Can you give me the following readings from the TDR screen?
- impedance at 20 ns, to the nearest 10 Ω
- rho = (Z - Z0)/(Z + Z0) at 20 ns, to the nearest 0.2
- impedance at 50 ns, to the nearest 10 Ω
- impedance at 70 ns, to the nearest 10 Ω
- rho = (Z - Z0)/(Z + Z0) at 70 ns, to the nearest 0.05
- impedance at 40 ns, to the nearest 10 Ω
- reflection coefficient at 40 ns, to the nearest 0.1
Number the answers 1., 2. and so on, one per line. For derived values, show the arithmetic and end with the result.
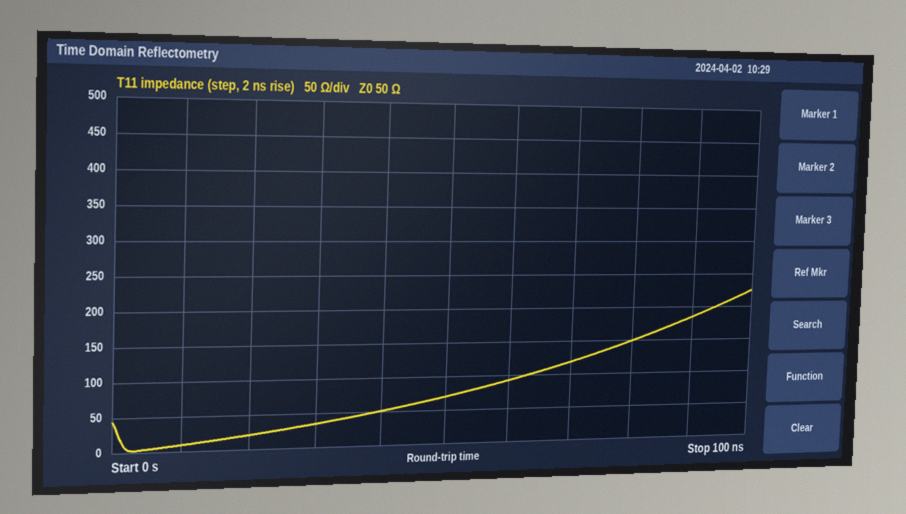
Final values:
1. 20 Ω
2. (20 − 50)/(20 + 50) ≈ -0.4
3. 70 Ω
4. 120 Ω
5. (120 − 50)/(120 + 50) ≈ +0.412, so +0.40 to the nearest 0.05
6. 50 Ω
7. (50 − 50)/(50 + 50) ≈ 0.0
